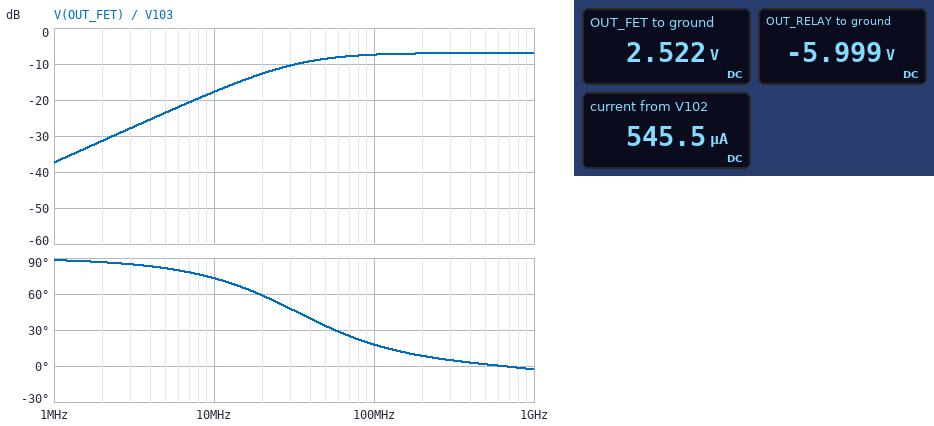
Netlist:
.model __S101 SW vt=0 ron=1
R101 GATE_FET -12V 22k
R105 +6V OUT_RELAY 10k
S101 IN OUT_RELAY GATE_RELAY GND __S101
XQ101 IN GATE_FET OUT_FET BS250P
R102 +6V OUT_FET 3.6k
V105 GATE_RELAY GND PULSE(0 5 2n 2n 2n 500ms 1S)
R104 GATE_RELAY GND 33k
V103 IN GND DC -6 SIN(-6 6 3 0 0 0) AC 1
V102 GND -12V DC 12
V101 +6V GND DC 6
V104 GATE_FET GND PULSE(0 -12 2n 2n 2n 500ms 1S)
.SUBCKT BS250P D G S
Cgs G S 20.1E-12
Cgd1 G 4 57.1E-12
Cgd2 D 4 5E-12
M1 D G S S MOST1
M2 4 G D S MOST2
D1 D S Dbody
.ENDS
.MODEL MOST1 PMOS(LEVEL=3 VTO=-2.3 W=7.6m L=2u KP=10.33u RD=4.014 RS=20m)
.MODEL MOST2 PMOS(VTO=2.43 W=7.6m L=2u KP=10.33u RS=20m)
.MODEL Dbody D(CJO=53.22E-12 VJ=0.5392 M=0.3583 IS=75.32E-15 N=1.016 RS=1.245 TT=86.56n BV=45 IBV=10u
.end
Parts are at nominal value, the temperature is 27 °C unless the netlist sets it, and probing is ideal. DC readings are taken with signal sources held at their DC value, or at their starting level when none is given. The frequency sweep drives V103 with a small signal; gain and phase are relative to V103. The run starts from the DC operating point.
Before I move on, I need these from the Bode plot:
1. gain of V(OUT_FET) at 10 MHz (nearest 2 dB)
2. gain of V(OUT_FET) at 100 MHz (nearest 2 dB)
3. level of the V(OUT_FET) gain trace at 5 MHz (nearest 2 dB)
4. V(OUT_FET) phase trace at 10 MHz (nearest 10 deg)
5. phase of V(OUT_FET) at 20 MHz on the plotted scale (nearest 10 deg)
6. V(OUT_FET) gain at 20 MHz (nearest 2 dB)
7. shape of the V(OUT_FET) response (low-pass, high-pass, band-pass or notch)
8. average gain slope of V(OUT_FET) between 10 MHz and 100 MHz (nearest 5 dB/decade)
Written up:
-18 dB
-8 dB
-24 dB
70 deg
60 deg
-12 dB
high-pass
10 dB/decade
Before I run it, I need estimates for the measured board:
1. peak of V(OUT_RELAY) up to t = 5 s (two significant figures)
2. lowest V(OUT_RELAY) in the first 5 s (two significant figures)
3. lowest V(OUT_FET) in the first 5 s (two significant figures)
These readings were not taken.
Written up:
6.0 V
-12 V
-9.2 V
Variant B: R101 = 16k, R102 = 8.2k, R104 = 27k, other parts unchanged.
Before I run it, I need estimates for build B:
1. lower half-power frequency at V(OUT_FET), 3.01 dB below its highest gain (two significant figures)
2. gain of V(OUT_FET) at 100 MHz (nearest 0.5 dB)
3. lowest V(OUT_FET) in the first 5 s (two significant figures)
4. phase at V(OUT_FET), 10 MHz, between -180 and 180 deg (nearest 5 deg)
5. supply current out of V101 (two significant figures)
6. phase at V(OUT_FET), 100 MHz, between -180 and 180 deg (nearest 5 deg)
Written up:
22 MHz
-7.0 dB
-9.4 V
65 deg
1.6 mA
10 deg
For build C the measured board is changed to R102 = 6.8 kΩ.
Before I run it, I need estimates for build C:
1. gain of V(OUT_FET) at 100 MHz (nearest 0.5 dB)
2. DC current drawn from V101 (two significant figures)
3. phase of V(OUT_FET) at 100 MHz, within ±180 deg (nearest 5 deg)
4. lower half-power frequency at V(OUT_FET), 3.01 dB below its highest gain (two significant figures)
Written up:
-7.0 dB
1.7 mA
15 deg
24 MHz
